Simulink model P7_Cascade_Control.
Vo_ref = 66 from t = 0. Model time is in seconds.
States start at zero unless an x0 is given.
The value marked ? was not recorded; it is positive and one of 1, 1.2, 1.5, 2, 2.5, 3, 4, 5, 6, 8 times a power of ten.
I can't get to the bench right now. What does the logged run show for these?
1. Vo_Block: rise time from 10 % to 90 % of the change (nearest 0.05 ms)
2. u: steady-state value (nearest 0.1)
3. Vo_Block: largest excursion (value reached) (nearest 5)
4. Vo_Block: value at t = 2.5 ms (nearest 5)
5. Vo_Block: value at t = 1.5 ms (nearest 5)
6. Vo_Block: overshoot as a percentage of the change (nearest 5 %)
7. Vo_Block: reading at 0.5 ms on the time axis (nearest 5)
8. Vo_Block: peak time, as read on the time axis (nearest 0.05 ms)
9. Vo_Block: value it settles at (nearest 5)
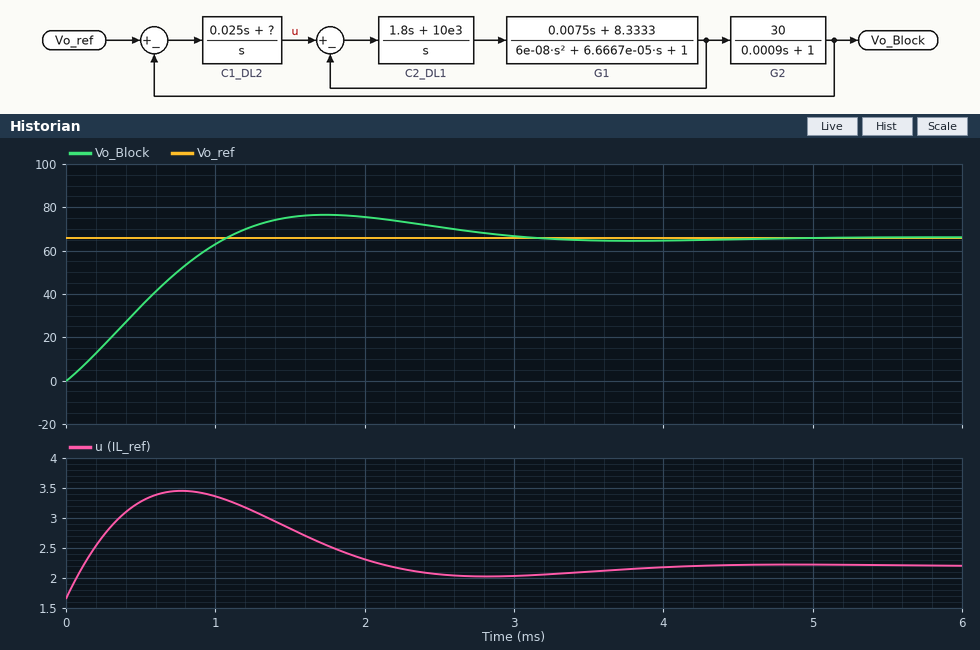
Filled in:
0.80 ms
2.2
75
70
75
15 %
35
1.75 ms
65
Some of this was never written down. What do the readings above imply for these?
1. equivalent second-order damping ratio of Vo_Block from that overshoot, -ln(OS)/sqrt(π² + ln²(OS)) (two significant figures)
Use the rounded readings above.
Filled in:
0.52
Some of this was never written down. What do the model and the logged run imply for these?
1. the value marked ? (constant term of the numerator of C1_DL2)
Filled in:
100
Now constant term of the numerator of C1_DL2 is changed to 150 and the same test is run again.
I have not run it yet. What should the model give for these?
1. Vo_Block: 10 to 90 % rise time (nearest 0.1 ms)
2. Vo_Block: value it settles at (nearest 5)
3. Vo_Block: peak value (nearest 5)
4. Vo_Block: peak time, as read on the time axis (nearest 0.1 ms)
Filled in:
0.6 ms
65
80
1.4 ms
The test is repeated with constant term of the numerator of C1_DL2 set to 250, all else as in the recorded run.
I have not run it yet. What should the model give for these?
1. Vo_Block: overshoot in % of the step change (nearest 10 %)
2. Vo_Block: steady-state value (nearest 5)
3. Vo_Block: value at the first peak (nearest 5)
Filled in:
30 %
65
90
